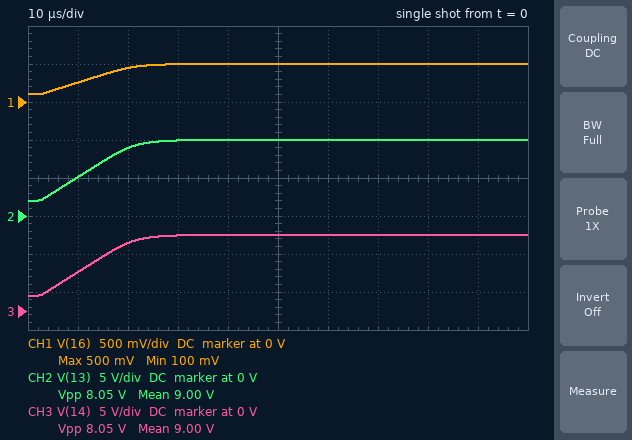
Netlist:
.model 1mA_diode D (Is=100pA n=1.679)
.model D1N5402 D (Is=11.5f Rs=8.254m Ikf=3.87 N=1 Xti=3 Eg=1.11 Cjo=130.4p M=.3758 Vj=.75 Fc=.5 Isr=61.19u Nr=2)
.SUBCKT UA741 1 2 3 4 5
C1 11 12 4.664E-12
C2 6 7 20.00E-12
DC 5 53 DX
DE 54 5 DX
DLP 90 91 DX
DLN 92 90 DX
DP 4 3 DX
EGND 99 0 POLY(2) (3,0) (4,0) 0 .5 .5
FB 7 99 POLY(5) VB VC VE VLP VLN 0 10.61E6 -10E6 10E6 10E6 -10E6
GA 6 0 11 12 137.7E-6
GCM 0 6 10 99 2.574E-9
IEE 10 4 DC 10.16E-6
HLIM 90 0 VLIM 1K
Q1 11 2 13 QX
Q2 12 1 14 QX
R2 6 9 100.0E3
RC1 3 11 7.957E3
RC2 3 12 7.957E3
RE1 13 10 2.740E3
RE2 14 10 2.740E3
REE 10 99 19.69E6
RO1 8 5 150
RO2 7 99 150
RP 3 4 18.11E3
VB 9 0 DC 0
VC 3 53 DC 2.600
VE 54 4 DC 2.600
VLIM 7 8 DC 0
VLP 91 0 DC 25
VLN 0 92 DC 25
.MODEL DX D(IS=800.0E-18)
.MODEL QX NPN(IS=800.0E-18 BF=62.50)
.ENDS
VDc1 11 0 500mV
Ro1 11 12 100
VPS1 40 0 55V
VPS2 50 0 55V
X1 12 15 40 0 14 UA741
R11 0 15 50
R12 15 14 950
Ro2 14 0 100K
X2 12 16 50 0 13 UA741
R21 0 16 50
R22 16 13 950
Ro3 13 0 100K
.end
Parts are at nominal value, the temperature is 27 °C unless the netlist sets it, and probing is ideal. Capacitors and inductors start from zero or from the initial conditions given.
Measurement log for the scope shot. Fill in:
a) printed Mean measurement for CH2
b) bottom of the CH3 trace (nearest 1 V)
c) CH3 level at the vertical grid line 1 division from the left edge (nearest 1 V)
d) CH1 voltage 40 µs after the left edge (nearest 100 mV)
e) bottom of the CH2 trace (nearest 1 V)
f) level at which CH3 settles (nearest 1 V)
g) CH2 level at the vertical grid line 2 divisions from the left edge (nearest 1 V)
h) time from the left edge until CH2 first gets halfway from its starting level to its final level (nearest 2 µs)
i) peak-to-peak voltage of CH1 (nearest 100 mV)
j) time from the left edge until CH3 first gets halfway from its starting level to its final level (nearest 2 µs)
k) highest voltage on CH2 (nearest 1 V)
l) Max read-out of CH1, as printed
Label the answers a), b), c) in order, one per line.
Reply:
a) 9.00 V
b) 2 V
c) 5 V
d) 500 mV
e) 2 V
f) 10 V
g) 9 V
h) 12 µs
i) 400 mV
j) 12 µs
k) 10 V
l) 500 mV
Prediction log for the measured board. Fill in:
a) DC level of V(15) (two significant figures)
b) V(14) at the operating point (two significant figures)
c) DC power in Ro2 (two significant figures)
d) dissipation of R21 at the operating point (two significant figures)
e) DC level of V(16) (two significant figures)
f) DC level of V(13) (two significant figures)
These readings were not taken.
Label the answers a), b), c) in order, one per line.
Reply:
a) 500 mV
b) 10 V
c) 1.0 mW
d) 5.0 mW
e) 500 mV
f) 10 V
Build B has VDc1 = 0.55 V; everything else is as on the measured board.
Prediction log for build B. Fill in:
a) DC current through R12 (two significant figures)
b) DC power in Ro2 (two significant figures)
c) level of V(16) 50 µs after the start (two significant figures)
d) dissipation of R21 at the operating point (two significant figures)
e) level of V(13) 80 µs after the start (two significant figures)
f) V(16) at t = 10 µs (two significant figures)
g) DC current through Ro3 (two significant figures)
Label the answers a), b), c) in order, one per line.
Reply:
a) 11 mA
b) 1.2 mW
c) 550 mV
d) 6.1 mW
e) 11 V
f) 260 mV
g) 110 µA
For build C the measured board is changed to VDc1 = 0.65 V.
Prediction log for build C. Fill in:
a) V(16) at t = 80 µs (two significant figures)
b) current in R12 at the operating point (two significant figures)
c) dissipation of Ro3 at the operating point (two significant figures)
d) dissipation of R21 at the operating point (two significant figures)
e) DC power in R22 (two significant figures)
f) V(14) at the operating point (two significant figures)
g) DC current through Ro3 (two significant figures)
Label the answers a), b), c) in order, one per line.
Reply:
a) 650 mV
b) 13 mA
c) 1.7 mW
d) 8.5 mW
e) 160 mW
f) 13 V
g) 130 µA
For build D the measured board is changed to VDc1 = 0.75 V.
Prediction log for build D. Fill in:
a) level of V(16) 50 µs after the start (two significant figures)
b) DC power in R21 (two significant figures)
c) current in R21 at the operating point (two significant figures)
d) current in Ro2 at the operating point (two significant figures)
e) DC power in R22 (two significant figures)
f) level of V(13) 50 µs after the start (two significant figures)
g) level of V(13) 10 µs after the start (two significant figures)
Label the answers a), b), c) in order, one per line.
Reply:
a) 750 mV
b) 11 mW
c) 15 mA
d) 150 µA
e) 210 mW
f) 15 V
g) 5.1 V
